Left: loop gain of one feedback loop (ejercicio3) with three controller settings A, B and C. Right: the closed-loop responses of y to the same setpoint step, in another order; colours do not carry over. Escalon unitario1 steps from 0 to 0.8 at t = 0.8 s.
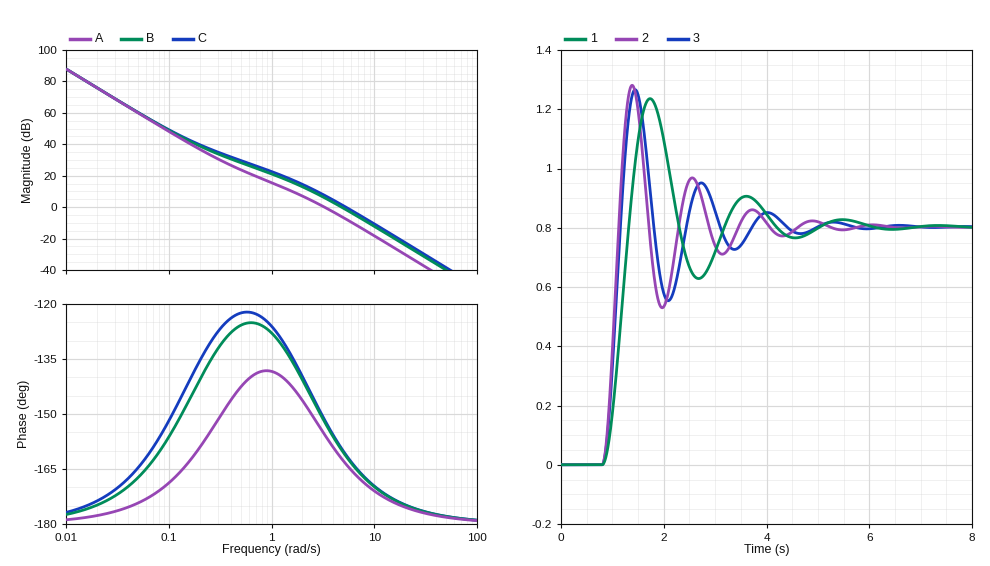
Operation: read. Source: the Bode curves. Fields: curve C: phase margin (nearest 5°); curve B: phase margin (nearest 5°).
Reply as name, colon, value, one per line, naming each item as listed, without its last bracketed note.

curve C: phase margin: 20°
curve B: phase margin: 20°
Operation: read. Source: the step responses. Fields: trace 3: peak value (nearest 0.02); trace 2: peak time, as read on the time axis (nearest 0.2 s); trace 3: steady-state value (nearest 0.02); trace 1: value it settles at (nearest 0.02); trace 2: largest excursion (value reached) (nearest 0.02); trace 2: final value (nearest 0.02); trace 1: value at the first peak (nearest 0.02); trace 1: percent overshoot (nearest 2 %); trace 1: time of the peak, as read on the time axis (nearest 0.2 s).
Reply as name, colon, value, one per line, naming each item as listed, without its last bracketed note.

trace 3: peak value: 1.26
trace 2: peak time, as read on the time axis: 1.4 s
trace 3: steady-state value: 0.80
trace 1: value it settles at: 0.80
trace 2: largest excursion (value reached): 1.28
trace 2: final value: 0.80
trace 1: value at the first peak: 1.24
trace 1: percent overshoot: 54 %
trace 1: time of the peak, as read on the time axis: 1.8 s
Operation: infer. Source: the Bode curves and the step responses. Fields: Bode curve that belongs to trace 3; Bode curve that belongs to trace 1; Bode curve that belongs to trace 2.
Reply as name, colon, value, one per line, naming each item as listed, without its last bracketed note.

Bode curve that belongs to trace 3: B
Bode curve that belongs to trace 1: A
Bode curve that belongs to trace 2: C
